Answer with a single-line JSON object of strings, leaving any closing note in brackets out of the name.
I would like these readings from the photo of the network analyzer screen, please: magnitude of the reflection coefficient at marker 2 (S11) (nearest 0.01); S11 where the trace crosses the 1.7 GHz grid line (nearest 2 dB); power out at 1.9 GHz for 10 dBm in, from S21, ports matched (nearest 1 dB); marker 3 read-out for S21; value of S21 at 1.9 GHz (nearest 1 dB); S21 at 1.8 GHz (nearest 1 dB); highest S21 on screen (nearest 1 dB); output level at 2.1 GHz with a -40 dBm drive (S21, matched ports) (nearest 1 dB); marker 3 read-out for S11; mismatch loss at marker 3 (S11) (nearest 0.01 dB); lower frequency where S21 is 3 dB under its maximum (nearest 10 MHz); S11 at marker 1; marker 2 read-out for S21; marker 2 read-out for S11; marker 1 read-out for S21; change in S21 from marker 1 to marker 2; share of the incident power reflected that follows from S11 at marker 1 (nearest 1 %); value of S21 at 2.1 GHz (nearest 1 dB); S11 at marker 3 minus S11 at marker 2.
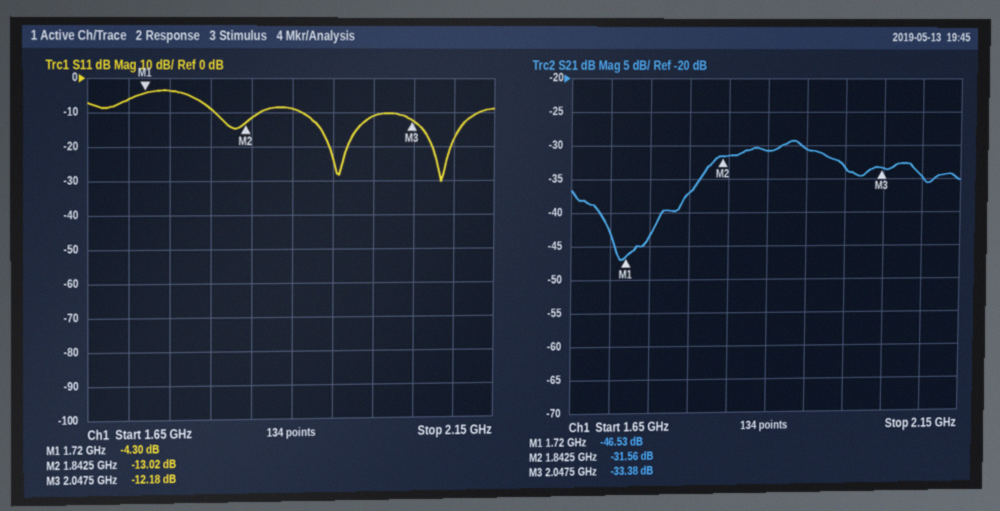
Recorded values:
{"magnitude of the reflection coefficient at marker 2 (S11)": "0.22", "S11 where the trace crosses the 1.7 GHz grid line": "-6 dB", "power out at 1.9 GHz for 10 dBm in, from S21, ports matched": "-21 dBm", "marker 3 read-out for S21": "-33.38 dB", "value of S21 at 1.9 GHz": "-31 dB", "S21 at 1.8 GHz": "-37 dB", "highest S21 on screen": "-29 dB", "output level at 2.1 GHz with a -40 dBm drive (S21, matched ports)": "-75 dBm", "marker 3 read-out for S11": "-12.18 dB", "mismatch loss at marker 3 (S11)": "0.27 dB", "lower frequency where S21 is 3 dB under its maximum": "1.83 GHz", "S11 at marker 1": "-4.30 dB", "marker 2 read-out for S21": "-31.56 dB", "marker 2 read-out for S11": "-13.02 dB", "marker 1 read-out for S21": "-46.53 dB", "change in S21 from marker 1 to marker 2": "14.97 dB", "share of the incident power reflected that follows from S11 at marker 1": "37 %", "value of S21 at 2.1 GHz": "-35 dB", "S11 at marker 3 minus S11 at marker 2": "0.84 dB"}
